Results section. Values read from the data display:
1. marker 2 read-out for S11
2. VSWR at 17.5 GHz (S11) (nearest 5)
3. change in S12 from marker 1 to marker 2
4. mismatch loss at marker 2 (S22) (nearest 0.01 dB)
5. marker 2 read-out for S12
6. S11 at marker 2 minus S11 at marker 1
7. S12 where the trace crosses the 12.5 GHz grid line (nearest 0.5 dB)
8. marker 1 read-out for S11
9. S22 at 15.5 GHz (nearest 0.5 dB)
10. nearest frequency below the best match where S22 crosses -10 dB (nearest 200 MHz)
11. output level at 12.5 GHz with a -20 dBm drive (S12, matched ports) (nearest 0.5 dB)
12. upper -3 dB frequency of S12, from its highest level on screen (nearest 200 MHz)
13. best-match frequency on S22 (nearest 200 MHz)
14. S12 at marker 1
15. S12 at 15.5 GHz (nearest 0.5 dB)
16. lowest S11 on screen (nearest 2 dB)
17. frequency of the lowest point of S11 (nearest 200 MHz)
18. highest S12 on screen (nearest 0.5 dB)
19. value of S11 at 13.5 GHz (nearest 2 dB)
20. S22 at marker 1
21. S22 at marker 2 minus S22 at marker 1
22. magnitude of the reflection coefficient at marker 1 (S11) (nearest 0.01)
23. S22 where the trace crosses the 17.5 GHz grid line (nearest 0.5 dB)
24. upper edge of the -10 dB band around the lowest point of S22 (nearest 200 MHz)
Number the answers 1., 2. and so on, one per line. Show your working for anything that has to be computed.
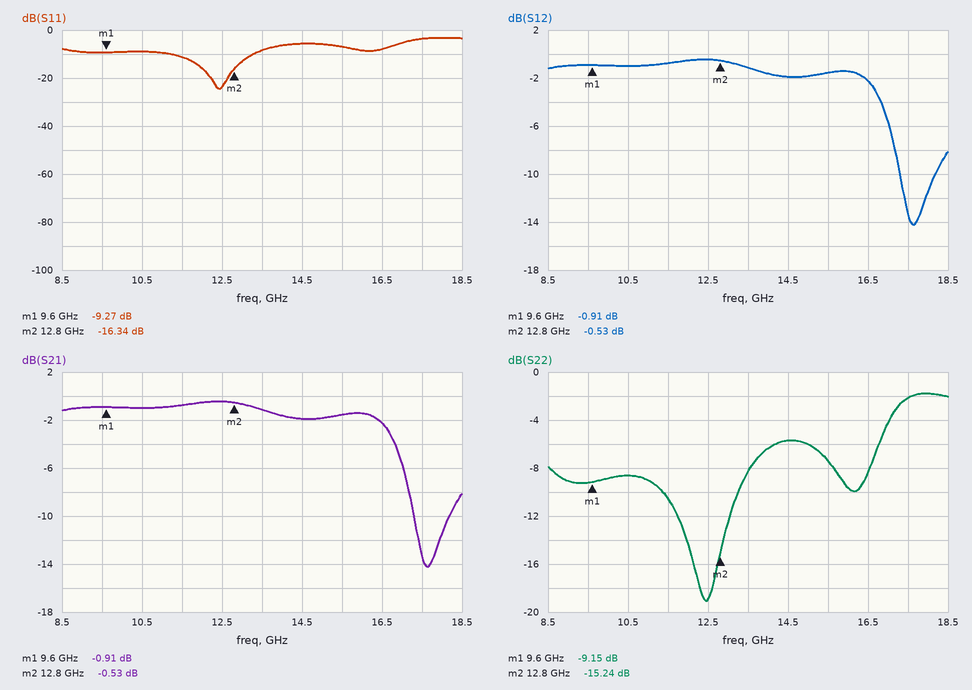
1. -16.34 dB
2. |Γ| = 10^(-4/20) = 0.6310; VSWR = (1 + 0.6310)/(1 − 0.6310) ≈ 4.42, so 5 to the nearest 5
3. -0.53 − (-0.91) = 0.38 dB
4. −10 log10(1 − 10^(-15.24/10)) ≈ 0.13 dB
5. -0.53 dB
6. -16.34 − (-9.27) = -7.07 dB
7. -0.5 dB
8. -9.27 dB
9. -7.5 dB
10. 11.4 GHz
11. -20 dBm + (-0.5 dB) = -20.5 dBm
12. 16.8 GHz
13. 12.4 GHz
14. -0.91 dB
15. -1.5 dB
16. -24 dB
17. 12.4 GHz
18. -0.5 dB
19. -8 dB
20. -9.15 dB
21. -15.24 − (-9.15) = -6.09 dB
22. 10^(-9.27/20) ≈ 0.34
23. -2.0 dB
24. 13.2 GHz
